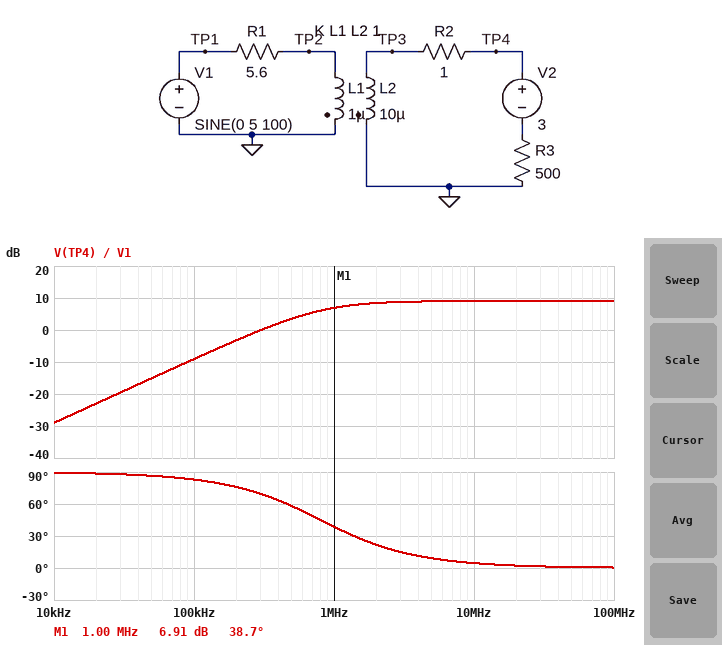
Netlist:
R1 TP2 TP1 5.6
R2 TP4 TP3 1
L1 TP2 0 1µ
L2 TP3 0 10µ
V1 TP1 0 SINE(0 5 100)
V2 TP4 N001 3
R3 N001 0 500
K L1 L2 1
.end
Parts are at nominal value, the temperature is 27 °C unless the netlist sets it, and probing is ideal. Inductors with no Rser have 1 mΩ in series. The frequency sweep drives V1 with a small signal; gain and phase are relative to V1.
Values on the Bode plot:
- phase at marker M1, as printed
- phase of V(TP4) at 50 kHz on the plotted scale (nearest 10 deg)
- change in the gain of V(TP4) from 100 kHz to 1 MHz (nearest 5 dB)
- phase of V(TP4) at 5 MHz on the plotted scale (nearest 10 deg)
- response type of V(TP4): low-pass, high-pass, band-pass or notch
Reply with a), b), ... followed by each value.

a) 38.7 deg
b) 90 deg
c) 15 dB
d) 10 deg
e) high-pass
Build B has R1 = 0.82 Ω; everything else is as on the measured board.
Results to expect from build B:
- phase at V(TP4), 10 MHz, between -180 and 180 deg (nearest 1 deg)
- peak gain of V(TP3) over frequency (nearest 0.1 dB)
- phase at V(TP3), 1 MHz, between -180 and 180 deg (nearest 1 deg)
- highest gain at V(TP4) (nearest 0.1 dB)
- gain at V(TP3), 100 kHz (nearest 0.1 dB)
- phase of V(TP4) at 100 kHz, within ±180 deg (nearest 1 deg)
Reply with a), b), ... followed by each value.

a) 1 deg
b) 9.9 dB
c) 7 deg
d) 9.8 dB
e) 5.6 dB
f) 52 deg
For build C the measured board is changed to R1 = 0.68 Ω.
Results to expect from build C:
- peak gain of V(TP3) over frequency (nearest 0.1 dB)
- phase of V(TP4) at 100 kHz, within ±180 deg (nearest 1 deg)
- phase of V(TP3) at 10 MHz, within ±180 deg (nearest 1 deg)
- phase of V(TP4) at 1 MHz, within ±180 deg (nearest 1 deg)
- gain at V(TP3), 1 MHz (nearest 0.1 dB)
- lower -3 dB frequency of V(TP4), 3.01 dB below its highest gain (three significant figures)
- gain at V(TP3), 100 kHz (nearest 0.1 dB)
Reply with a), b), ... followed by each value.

a) 9.9 dB
b) 47 deg
c) 1 deg
d) 6 deg
e) 9.8 dB
f) 107 kHz
g) 6.6 dB
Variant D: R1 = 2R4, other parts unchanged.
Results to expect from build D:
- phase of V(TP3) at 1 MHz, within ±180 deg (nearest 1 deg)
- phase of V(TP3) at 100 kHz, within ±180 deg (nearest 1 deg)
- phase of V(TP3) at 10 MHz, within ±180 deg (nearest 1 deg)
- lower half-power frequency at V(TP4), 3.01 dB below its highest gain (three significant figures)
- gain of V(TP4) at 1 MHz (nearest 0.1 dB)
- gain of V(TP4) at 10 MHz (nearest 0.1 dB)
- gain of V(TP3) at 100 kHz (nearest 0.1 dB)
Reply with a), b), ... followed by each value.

a) 20 deg
b) 75 deg
c) 2 deg
d) 365 kHz
e) 9.0 dB
f) 9.6 dB
g) -2.0 dB
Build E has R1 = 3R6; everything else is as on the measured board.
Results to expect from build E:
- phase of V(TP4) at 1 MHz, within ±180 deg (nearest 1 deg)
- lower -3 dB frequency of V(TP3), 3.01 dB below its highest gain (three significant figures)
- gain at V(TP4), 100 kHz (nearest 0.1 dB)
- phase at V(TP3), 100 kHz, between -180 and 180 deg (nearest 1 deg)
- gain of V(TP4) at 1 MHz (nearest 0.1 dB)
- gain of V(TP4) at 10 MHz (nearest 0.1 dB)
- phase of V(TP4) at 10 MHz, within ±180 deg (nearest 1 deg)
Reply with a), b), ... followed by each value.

a) 28 deg
b) 535 kHz
c) -5.3 dB
d) 79 deg
e) 8.3 dB
f) 9.4 dB
g) 3 deg
